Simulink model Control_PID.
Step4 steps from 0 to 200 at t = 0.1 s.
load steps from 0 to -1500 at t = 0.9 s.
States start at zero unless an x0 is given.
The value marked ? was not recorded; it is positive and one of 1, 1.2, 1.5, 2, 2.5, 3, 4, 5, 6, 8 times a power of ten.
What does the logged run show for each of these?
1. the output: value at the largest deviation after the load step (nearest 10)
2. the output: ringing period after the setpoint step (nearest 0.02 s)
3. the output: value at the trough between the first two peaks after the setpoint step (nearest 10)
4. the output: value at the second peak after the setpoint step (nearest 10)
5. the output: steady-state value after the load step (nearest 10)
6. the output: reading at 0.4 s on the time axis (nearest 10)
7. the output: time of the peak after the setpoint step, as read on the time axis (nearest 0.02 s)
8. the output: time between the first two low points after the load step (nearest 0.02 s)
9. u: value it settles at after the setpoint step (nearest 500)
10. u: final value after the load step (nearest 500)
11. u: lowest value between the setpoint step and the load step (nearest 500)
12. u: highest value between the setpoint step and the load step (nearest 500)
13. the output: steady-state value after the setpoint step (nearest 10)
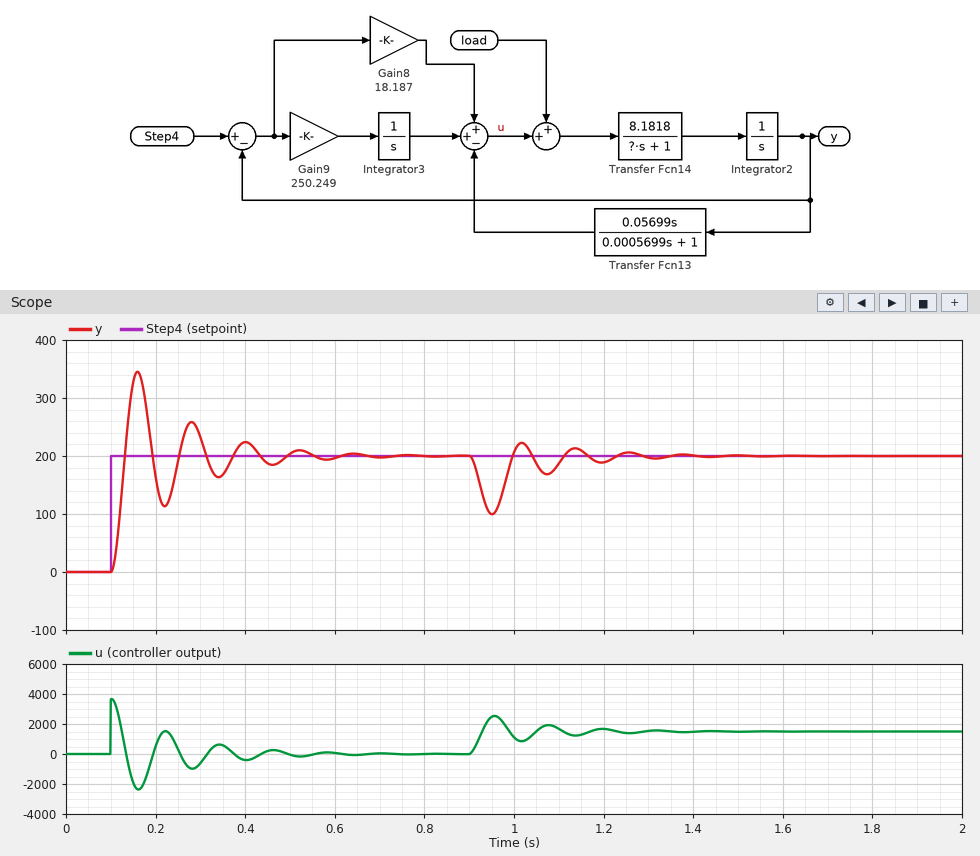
100
0.12 s
110
260
200
220
0.16 s
0.12 s
0
1500
-2500
3500
200
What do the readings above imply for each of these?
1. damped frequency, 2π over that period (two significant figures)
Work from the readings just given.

52 rad/s
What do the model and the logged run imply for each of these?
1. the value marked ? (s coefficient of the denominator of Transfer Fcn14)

0.05
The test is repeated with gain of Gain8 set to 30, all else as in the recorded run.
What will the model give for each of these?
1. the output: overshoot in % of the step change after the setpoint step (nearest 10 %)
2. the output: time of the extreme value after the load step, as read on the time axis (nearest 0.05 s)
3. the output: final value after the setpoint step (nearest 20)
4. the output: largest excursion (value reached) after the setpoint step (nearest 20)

70 %
0.95 s
200
340
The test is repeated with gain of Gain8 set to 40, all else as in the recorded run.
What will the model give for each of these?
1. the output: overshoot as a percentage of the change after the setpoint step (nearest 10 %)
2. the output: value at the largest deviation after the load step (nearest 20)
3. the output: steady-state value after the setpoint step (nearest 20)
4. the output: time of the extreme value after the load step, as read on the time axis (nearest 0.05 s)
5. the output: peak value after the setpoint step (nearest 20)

70 %
140
200
0.95 s
340
